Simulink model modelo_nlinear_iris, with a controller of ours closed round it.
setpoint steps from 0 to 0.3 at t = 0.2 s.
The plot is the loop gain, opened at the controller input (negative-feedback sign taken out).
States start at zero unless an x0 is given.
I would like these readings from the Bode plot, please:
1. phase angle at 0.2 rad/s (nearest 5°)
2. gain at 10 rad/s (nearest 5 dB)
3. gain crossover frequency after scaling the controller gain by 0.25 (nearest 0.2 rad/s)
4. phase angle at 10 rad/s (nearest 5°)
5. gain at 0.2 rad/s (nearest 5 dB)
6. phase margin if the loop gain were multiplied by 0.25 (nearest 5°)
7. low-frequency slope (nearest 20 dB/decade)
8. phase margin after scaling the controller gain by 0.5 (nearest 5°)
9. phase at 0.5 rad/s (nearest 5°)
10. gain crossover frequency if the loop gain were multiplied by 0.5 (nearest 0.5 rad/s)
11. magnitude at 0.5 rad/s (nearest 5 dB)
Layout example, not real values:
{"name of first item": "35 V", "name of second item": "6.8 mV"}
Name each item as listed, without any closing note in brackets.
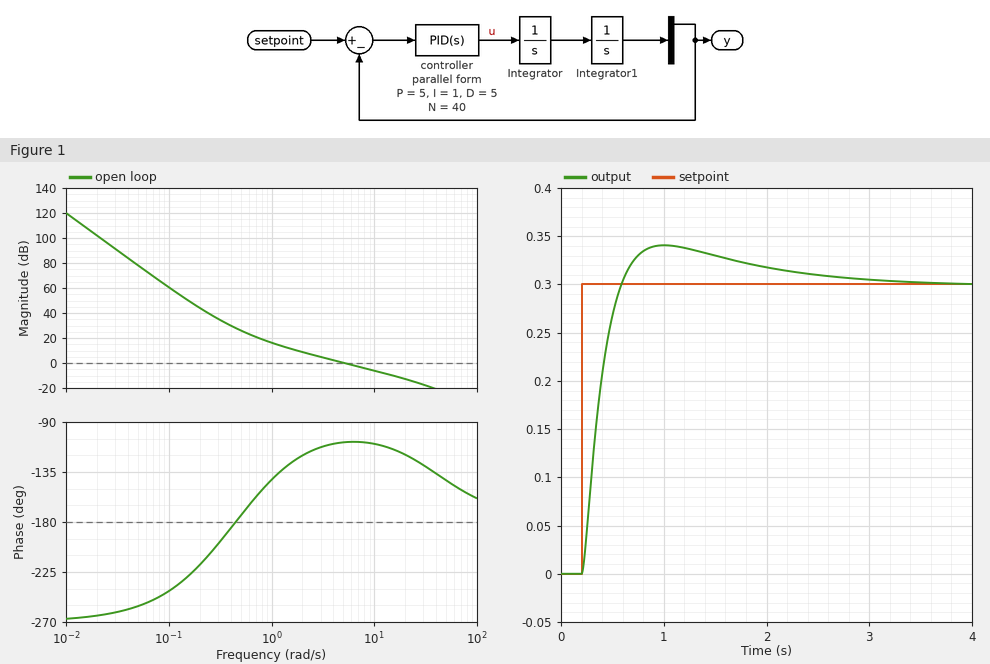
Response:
{"phase angle at 0.2 rad/s": "-220°", "gain at 10 rad/s": "-5 dB", "gain crossover frequency after scaling the controller gain by 0.25": "1.4 rad/s", "phase angle at 10 rad/s": "-110°", "gain at 0.2 rad/s": "45 dB", "phase margin if the loop gain were multiplied by 0.25": "50°", "low-frequency slope": "-60 dB/decade", "phase margin after scaling the controller gain by 0.5": "65°", "phase at 0.5 rad/s": "-175°", "gain crossover frequency if the loop gain were multiplied by 0.5": "2.5 rad/s", "magnitude at 0.5 rad/s": "25 dB"}
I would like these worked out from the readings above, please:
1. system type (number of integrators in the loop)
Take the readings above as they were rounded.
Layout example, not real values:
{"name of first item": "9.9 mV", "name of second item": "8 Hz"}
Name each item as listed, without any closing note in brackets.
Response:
{"system type": "3"}
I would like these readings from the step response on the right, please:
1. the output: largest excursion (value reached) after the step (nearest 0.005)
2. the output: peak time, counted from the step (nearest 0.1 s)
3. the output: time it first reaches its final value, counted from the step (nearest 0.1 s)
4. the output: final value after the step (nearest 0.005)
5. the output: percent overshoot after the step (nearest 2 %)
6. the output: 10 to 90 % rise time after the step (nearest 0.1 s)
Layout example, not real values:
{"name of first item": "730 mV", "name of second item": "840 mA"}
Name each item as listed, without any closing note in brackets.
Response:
{"the output: largest excursion (value reached) after the step": "0.340", "the output: peak time, counted from the step": "0.8 s", "the output: time it first reaches its final value, counted from the step": "0.4 s", "the output: final value after the step": "0.300", "the output: percent overshoot after the step": "14 %", "the output: 10 to 90 % rise time after the step": "0.3 s"}
